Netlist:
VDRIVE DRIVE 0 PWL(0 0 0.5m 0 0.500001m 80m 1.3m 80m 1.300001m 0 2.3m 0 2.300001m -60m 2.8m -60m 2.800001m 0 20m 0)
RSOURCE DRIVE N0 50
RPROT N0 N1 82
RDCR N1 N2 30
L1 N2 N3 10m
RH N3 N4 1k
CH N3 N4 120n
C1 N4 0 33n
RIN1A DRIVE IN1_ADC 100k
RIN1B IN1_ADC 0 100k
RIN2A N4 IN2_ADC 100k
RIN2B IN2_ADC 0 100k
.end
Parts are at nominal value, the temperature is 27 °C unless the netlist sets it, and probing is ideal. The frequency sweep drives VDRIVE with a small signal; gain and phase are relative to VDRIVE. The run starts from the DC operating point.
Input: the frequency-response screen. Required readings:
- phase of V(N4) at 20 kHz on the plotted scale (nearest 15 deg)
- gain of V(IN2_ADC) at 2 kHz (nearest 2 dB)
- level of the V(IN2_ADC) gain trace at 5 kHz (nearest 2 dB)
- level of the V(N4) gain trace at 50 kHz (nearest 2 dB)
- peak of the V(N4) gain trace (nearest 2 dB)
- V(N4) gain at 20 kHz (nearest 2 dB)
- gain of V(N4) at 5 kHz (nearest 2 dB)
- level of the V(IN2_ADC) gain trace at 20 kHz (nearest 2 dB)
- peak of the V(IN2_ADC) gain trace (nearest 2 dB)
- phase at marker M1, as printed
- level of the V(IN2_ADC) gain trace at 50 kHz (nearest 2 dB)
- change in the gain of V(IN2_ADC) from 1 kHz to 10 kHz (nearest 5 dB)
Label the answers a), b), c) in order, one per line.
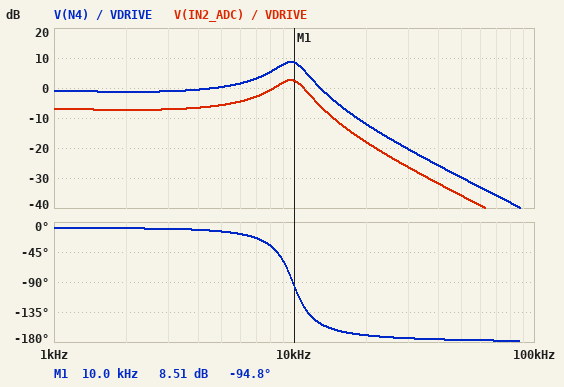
a) -165 deg
b) -8 dB
c) -6 dB
d) -30 dB
e) 8 dB
f) -12 dB
g) 0 dB
h) -18 dB
i) 2 dB
j) -94.8 deg
k) -36 dB
l) 10 dB
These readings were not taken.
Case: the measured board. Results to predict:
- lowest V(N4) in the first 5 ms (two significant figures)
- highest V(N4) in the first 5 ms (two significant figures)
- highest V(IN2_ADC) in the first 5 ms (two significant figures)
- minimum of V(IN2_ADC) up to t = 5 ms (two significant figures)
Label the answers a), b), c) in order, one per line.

a) -80 mV
b) 110 mV
c) 53 mV
d) -40 mV
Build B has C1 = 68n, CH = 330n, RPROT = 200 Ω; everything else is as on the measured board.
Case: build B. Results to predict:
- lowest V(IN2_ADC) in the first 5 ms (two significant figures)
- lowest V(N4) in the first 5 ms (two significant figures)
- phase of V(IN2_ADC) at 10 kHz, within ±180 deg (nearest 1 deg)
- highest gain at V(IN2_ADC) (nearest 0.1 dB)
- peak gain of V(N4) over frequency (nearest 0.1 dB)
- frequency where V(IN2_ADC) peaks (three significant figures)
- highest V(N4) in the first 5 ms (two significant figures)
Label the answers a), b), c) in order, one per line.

a) -33 mV
b) -66 mV
c) -141 deg
d) -3.8 dB
e) 2.2 dB
f) 5.91 kHz
g) 89 mV
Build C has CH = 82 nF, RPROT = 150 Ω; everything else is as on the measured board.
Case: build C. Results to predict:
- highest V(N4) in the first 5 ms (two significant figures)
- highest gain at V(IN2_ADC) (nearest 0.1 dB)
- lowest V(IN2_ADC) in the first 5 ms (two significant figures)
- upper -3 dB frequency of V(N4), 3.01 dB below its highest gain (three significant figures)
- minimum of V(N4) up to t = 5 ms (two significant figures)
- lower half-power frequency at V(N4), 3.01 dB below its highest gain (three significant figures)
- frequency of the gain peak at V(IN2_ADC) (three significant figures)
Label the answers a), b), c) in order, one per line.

a) 93 mV
b) -1.0 dB
c) -35 mV
d) 12.0 kHz
e) -70 mV
f) 7.48 kHz
g) 9.99 kHz
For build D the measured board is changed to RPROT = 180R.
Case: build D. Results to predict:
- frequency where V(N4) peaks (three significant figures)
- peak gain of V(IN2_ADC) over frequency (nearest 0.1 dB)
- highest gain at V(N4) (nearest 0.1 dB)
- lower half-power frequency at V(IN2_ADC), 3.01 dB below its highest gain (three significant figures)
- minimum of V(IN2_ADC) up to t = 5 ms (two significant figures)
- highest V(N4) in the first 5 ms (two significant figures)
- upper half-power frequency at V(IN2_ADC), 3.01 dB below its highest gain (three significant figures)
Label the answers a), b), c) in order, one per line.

a) 9.43 kHz
b) -1.0 dB
c) 5.0 dB
d) 6.75 kHz
e) -36 mV
f) 97 mV
g) 11.5 kHz
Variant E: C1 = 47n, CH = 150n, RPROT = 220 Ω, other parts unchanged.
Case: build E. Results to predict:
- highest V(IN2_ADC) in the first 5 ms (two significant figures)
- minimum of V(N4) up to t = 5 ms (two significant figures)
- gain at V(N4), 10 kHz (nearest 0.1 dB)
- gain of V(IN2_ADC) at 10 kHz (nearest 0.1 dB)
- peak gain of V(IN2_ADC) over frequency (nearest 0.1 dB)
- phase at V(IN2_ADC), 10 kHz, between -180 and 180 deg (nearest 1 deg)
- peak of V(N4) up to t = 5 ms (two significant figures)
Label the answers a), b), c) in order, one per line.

a) 43 mV
b) -65 mV
c) -0.6 dB
d) -6.6 dB
e) -3.6 dB
f) -121 deg
g) 87 mV
